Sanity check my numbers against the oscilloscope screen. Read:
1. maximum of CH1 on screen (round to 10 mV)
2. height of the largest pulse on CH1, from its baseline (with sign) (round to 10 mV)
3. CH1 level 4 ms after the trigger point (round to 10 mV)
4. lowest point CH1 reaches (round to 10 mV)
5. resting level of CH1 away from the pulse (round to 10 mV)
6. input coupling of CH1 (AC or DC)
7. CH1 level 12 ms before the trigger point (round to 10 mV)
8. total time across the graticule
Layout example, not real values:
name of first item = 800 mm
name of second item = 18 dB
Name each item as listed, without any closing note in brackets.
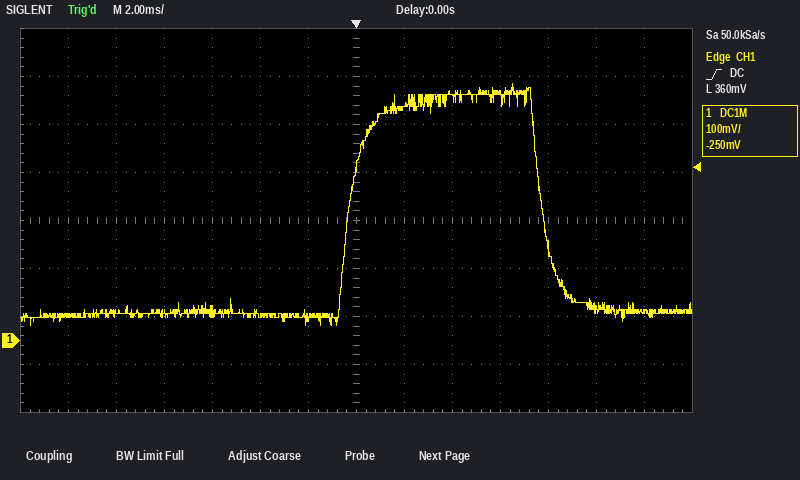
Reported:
maximum of CH1 on screen = 540 mV
height of the largest pulse on CH1, from its baseline (with sign) = +480 mV
CH1 level 4 ms after the trigger point = 500 mV
lowest point CH1 reaches = 30 mV
resting level of CH1 away from the pulse = 60 mV
input coupling of CH1 = DC
CH1 level 12 ms before the trigger point = 50 mV
total time across the graticule = 28 ms
